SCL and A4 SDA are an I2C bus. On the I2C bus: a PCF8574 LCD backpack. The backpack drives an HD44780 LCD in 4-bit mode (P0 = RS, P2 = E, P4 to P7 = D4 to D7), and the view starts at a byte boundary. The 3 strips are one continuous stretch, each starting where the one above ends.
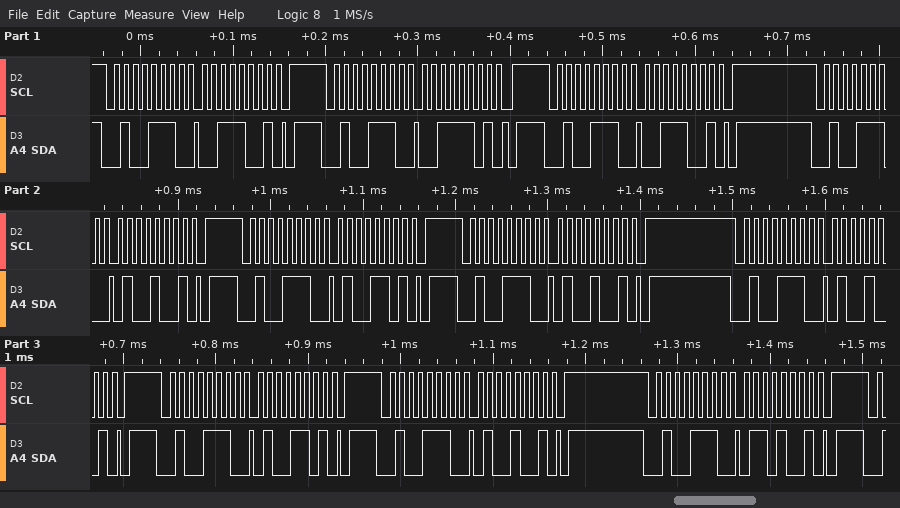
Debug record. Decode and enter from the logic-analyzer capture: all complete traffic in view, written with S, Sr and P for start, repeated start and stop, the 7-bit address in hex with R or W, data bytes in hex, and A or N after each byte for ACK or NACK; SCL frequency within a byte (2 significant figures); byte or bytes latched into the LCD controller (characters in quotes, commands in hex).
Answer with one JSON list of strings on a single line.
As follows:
["S 27W A 39 A P S 27W A 3D A P S 27W A 39 A P S 27W A 49 A P S 27W A 4D A P S 27W A 49 A P S 27W A 49 A P S 27W A 4D A P S 27W A 49 A P S 27W A 69 A P", "100 kHz", "'4'"]
